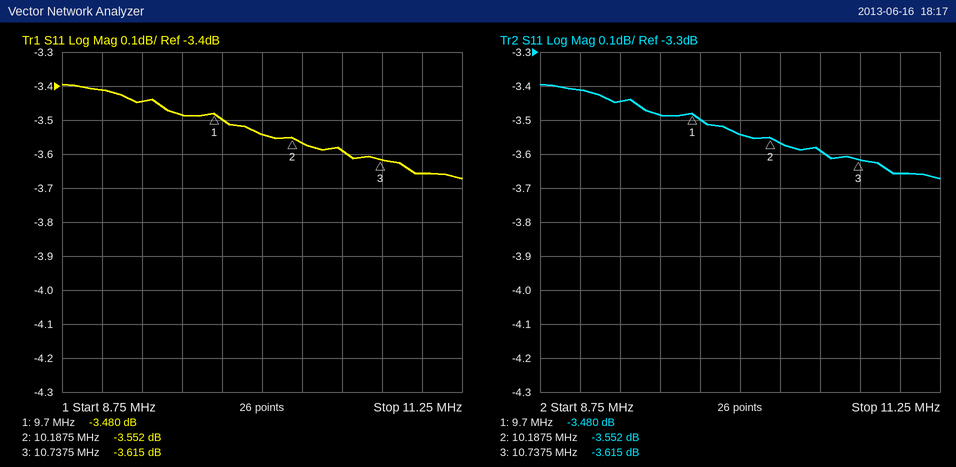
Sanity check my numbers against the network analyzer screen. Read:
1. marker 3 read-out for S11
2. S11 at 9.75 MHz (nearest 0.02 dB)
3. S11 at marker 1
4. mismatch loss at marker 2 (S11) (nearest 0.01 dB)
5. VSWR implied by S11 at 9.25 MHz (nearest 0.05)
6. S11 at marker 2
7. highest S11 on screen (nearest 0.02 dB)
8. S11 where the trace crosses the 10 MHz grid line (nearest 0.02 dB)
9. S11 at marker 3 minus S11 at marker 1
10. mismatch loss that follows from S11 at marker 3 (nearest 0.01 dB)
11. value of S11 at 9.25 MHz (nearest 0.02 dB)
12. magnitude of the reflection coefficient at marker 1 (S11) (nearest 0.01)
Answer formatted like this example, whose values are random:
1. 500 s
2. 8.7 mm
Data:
1. -3.615 dB
2. -3.50 dB
3. -3.480 dB
4. 2.53 dB
5. 5.10
6. -3.552 dB
7. -3.40 dB
8. -3.54 dB
9. -0.135 dB
10. 2.48 dB
11. -3.44 dB
12. 0.67
